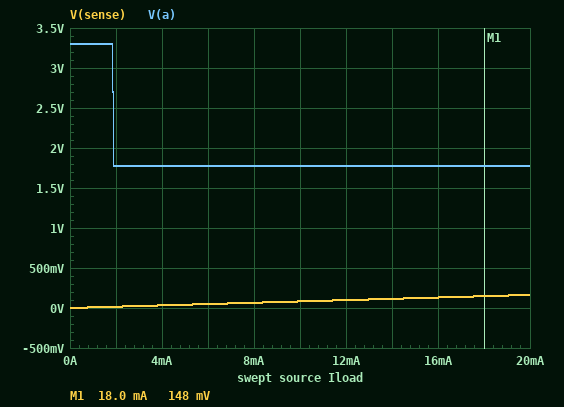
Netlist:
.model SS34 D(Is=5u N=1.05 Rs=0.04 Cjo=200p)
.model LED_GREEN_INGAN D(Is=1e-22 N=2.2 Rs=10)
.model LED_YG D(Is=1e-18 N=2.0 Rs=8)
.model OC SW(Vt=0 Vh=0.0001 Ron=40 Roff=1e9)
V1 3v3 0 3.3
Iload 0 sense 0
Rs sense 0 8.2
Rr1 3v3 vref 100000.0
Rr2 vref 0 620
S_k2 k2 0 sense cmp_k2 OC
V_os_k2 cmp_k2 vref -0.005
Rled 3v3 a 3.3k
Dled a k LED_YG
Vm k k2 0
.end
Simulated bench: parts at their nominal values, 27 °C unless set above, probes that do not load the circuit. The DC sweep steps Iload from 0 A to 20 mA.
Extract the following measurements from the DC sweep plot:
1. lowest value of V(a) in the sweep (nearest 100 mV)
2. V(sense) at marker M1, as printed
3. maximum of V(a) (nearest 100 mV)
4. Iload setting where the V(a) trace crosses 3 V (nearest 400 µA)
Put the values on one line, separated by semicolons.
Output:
1.8 V; 148 mV; 3.3 V; 2.0 mA
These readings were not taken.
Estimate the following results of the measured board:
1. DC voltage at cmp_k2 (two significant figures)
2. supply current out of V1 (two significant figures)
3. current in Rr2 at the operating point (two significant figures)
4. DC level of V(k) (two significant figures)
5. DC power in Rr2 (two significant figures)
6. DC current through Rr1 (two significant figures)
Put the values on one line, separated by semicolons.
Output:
15 mV; 33 µA; 33 µA; 2.2 V; 670 nW; 33 µA
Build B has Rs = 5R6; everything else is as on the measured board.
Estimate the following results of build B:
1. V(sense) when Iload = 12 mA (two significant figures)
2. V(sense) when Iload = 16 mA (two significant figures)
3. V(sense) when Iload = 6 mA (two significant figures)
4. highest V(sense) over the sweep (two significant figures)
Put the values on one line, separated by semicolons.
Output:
67 mV; 90 mV; 34 mV; 110 mV
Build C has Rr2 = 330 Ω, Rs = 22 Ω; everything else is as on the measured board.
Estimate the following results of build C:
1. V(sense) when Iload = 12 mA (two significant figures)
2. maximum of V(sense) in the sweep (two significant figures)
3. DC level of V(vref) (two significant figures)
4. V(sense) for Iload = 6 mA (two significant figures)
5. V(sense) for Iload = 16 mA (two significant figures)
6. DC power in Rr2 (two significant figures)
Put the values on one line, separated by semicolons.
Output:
260 mV; 440 mV; 11 mV; 130 mV; 350 mV; 360 nW
